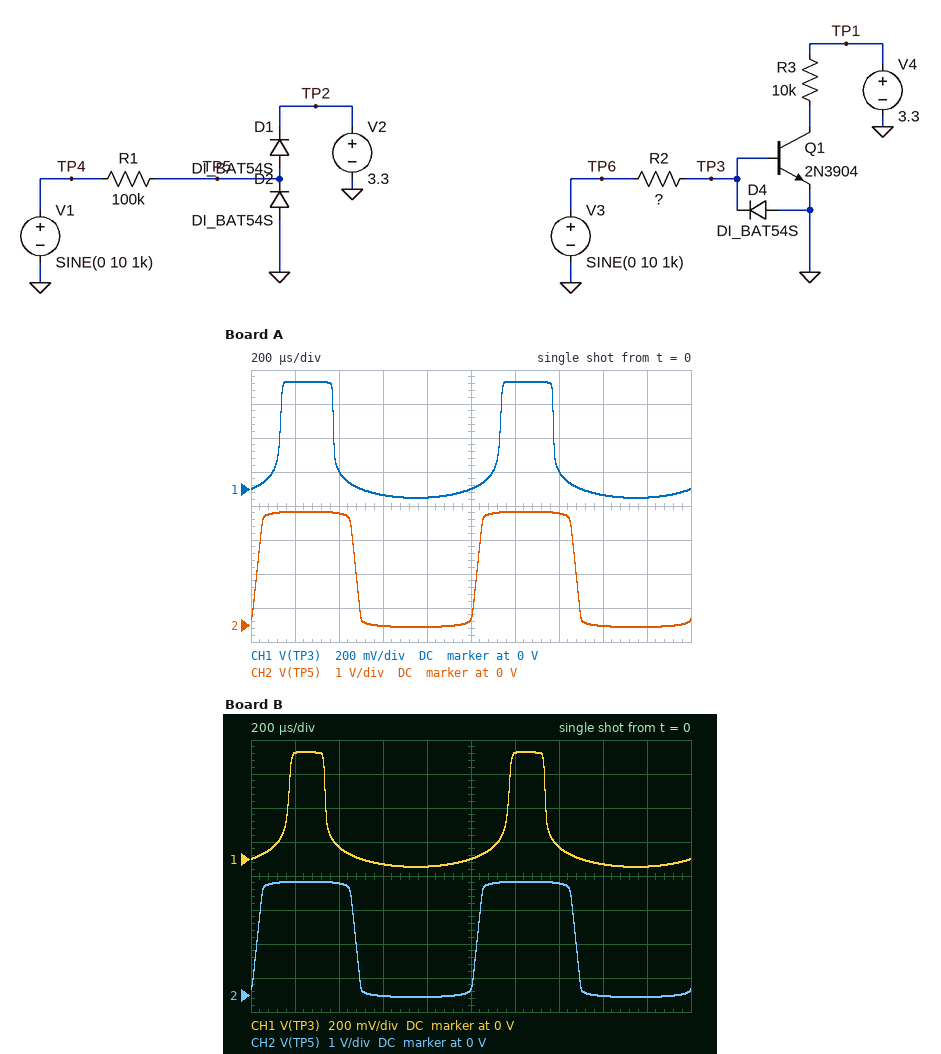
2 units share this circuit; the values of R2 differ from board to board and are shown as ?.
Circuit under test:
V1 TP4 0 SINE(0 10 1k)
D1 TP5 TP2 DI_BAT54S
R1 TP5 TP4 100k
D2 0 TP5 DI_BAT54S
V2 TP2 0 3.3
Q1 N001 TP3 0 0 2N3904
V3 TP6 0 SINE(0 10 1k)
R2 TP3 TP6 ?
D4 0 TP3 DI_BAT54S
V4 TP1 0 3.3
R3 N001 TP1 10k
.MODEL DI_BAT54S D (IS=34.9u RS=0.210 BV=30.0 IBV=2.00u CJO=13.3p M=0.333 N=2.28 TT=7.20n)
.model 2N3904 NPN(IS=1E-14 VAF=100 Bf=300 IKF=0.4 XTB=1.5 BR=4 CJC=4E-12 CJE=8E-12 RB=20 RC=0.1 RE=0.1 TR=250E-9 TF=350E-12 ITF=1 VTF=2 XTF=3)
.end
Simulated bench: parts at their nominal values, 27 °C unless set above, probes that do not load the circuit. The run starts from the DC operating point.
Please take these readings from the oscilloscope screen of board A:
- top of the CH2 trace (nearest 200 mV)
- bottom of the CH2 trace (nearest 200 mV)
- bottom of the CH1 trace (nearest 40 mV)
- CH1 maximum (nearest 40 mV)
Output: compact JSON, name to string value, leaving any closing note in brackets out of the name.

{"top of the CH2 trace": "3.4 V", "bottom of the CH2 trace": "0 V", "bottom of the CH1 trace": "-40 mV", "CH1 maximum": "640 mV"}
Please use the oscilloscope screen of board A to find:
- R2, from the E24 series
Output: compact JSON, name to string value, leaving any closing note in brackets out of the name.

{"R2, from the E24 series": "200 kΩ"}
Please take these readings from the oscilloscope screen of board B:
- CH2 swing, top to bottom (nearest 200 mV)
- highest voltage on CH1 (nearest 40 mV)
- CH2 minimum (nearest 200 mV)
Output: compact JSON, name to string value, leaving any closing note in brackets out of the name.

{"CH2 swing, top to bottom": "3.4 V", "highest voltage on CH1": "640 mV", "CH2 minimum": "0 V"}
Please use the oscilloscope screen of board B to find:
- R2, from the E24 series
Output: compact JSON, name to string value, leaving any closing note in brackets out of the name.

{"R2, from the E24 series": "240 kΩ"}
